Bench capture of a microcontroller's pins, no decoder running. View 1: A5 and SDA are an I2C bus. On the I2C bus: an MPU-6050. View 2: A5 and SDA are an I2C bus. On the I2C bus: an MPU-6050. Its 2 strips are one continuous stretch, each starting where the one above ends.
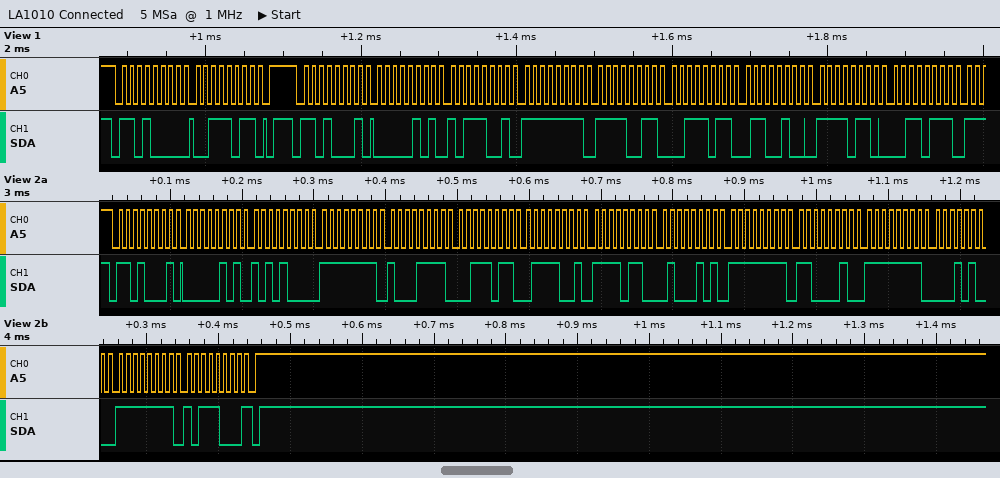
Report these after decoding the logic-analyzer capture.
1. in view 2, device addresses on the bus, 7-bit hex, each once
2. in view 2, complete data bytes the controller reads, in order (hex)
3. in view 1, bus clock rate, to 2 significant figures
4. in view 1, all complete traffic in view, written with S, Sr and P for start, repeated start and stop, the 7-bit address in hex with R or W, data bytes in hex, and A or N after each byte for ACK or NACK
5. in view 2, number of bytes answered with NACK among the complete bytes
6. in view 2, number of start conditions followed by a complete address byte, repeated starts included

0x68
05 A8 FF 8F 3B 79 F6 45 FF C2 FF 14 FF B8
100 kHz
S 68W A 3B A P S 68R A 05 A B9 A FF A F3 A 3B A 64 A F6 A 37 A
1
1
